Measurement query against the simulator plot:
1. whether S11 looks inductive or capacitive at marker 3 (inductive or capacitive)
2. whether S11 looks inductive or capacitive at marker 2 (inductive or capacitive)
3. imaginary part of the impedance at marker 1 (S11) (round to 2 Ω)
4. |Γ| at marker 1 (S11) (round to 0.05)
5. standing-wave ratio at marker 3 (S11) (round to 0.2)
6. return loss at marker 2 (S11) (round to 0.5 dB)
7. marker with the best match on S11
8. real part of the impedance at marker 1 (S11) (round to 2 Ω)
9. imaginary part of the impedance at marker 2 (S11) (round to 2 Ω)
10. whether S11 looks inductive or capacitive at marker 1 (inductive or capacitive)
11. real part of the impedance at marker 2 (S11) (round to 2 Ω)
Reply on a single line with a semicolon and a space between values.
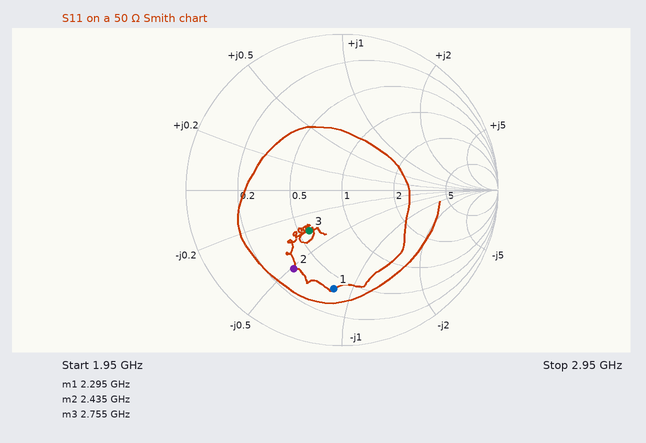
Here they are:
capacitive; capacitive; -42 Ω; 0.65; 2.0; 4.5 dB; marker 3; 20 Ω; -26 Ω; capacitive; 16 Ω
